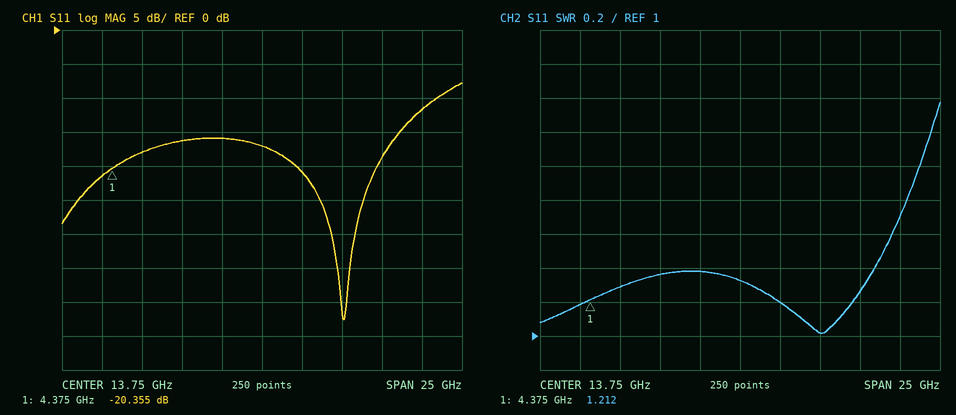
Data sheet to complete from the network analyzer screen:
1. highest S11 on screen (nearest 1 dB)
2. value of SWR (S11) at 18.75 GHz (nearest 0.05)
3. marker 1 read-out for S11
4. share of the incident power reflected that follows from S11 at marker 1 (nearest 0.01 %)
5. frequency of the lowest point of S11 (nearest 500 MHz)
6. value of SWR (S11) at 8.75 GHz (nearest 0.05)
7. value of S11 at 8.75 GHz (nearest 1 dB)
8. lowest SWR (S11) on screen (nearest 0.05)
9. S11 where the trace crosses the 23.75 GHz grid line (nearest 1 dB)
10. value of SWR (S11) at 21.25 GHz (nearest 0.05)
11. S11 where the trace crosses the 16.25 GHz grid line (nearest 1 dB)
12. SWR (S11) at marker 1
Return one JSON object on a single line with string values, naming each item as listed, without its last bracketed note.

{"highest S11 on screen": "-8 dB", "value of SWR (S11) at 18.75 GHz": "1.00", "marker 1 read-out for S11": "-20.355 dB", "share of the incident power reflected that follows from S11 at marker 1": "0.92 %", "frequency of the lowest point of S11": "19.0 GHz", "value of SWR (S11) at 8.75 GHz": "1.35", "value of S11 at 8.75 GHz": "-16 dB", "lowest SWR (S11) on screen": "1.00", "S11 where the trace crosses the 23.75 GHz grid line": "-12 dB", "value of SWR (S11) at 21.25 GHz": "1.25", "S11 where the trace crosses the 16.25 GHz grid line": "-21 dB", "SWR (S11) at marker 1": "1.212"}
